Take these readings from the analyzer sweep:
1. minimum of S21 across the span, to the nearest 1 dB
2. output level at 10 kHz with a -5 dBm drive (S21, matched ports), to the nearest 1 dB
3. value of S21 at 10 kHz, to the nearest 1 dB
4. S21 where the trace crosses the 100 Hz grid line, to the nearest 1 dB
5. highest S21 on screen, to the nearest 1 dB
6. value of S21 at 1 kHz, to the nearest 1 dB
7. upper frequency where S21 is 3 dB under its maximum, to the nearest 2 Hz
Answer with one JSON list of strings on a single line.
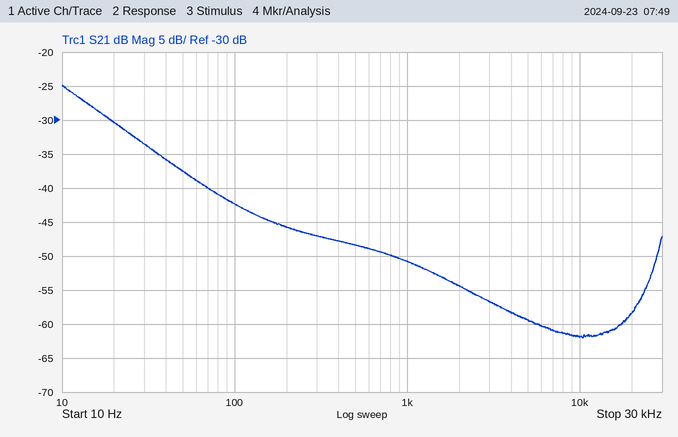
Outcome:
["-62 dB", "-67 dBm", "-62 dB", "-42 dB", "-25 dB", "-51 dB", "14 Hz"]
